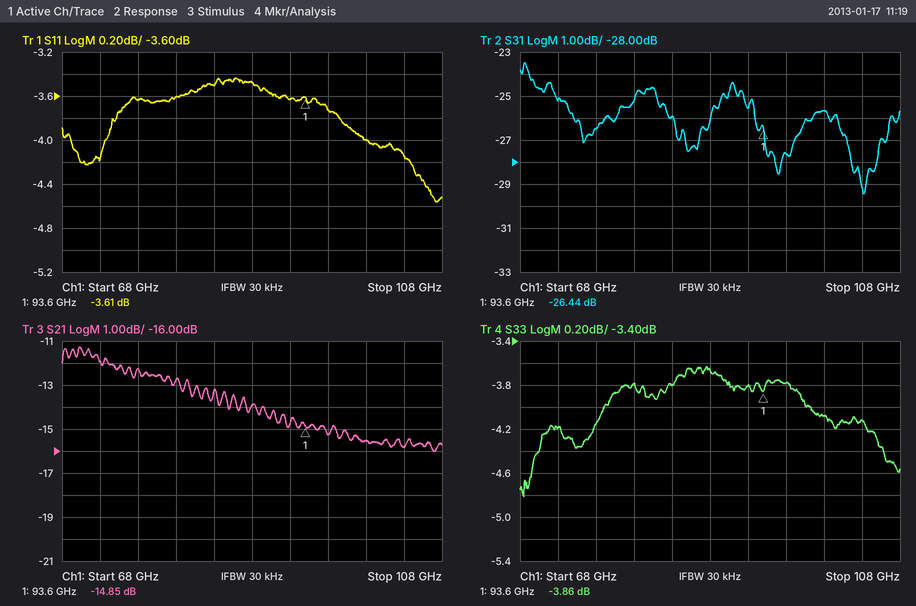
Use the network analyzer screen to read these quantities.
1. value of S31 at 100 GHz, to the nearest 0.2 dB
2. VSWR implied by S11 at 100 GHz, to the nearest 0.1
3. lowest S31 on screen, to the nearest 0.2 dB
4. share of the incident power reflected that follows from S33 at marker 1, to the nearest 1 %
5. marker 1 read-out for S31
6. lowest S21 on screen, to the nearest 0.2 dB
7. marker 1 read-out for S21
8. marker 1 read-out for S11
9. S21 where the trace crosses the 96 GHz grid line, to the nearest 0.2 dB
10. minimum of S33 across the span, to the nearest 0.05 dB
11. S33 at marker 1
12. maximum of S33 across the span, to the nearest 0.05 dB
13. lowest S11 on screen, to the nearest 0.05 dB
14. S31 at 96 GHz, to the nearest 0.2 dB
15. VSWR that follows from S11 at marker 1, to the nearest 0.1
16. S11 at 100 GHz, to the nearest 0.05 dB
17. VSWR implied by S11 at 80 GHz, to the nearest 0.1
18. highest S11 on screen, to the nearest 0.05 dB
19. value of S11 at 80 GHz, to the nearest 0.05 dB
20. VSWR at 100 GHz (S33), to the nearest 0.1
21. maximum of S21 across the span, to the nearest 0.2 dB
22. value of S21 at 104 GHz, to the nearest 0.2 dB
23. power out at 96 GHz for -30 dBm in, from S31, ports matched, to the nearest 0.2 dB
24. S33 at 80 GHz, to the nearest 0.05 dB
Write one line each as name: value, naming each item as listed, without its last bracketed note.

value of S31 at 100 GHz, to the nearest 0.2 dB: -25.6 dB
VSWR implied by S11 at 100 GHz, to the nearest 0.1: 4.4
lowest S31 on screen, to the nearest 0.2 dB: -29.4 dB
share of the incident power reflected that follows from S33 at marker 1, to the nearest 1 %: 41 %
marker 1 read-out for S31: -26.44 dB
lowest S21 on screen, to the nearest 0.2 dB: -16.0 dB
marker 1 read-out for S21: -14.85 dB
marker 1 read-out for S11: -3.61 dB
S21 where the trace crosses the 96 GHz grid line, to the nearest 0.2 dB: -15.2 dB
minimum of S33 across the span, to the nearest 0.05 dB: -4.80 dB
S33 at marker 1: -3.86 dB
maximum of S33 across the span, to the nearest 0.05 dB: -3.65 dB
lowest S11 on screen, to the nearest 0.05 dB: -4.55 dB
S31 at 96 GHz, to the nearest 0.2 dB: -27.6 dB
VSWR that follows from S11 at marker 1, to the nearest 0.1: 4.9
S11 at 100 GHz, to the nearest 0.05 dB: -4.00 dB
VSWR implied by S11 at 80 GHz, to the nearest 0.1: 4.9
highest S11 on screen, to the nearest 0.05 dB: -3.45 dB
value of S11 at 80 GHz, to the nearest 0.05 dB: -3.60 dB
VSWR at 100 GHz (S33), to the nearest 0.1: 4.3
maximum of S21 across the span, to the nearest 0.2 dB: -11.2 dB
value of S21 at 104 GHz, to the nearest 0.2 dB: -15.8 dB
power out at 96 GHz for -30 dBm in, from S31, ports matched, to the nearest 0.2 dB: -57.6 dBm
S33 at 80 GHz, to the nearest 0.05 dB: -3.80 dB
